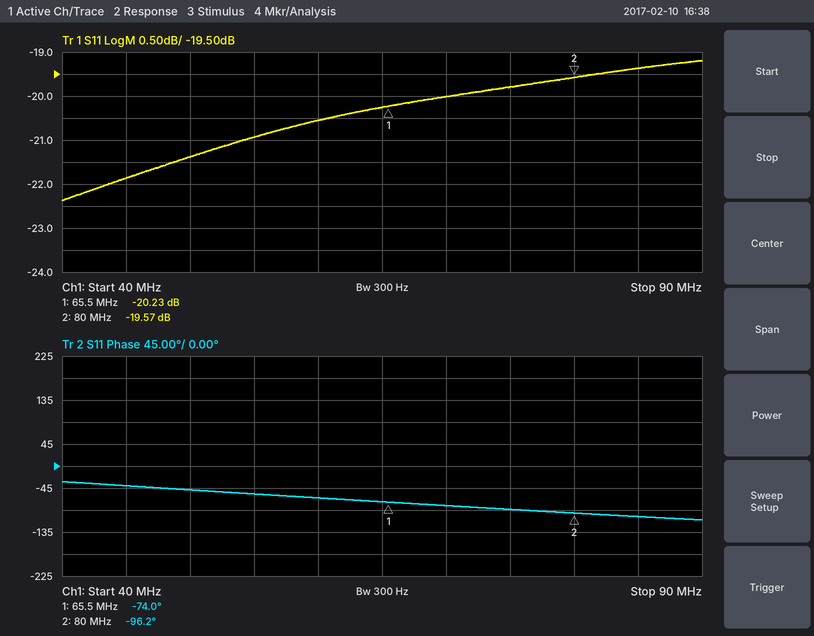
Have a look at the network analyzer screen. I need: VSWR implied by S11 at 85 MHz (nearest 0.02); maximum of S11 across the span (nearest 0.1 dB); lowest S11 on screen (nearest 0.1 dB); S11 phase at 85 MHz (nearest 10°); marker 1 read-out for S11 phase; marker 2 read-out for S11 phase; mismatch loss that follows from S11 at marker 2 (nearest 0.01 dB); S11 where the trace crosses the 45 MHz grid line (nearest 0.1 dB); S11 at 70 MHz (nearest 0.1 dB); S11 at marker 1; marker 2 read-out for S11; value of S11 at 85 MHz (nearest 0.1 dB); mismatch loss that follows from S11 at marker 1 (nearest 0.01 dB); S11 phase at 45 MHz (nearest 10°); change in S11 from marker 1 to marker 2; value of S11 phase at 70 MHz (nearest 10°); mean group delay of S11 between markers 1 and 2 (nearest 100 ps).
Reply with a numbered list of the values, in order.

1. 1.24
2. -19.2 dB
3. -22.4 dB
4. -100°
5. -74.0°
6. -96.2°
7. 0.05 dB
8. -21.9 dB
9. -20.0 dB
10. -20.23 dB
11. -19.57 dB
12. -19.4 dB
13. 0.04 dB
14. -40°
15. 0.66 dB
16. -80°
17. 4.3 ns
